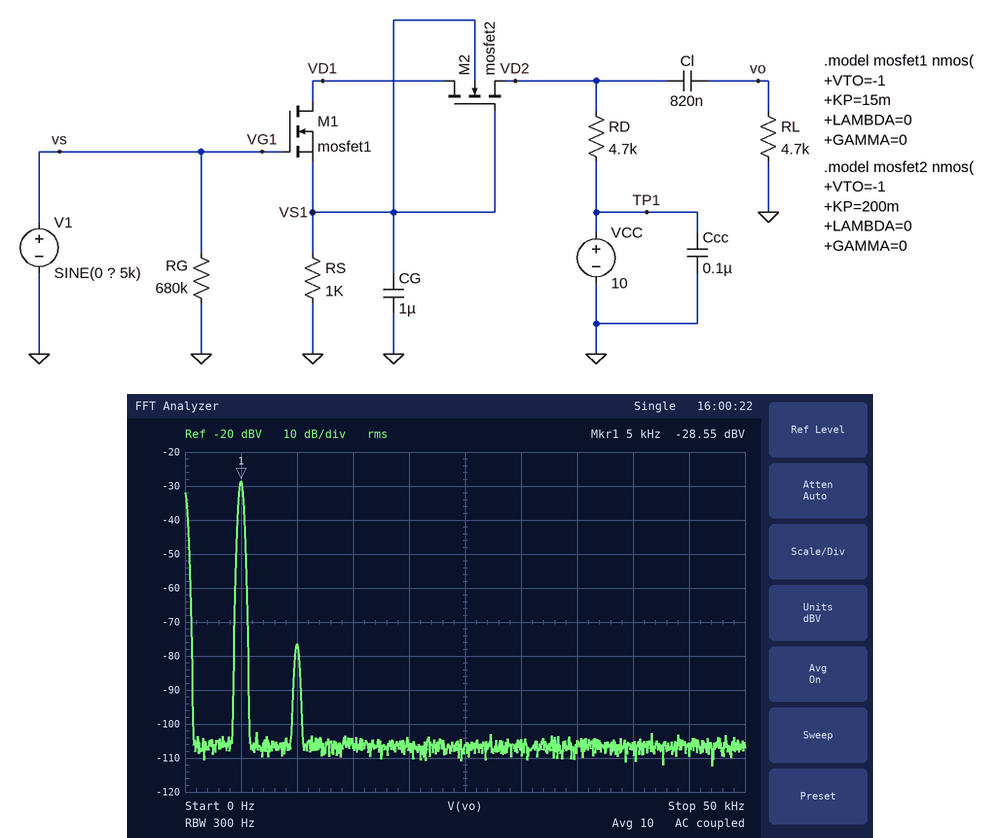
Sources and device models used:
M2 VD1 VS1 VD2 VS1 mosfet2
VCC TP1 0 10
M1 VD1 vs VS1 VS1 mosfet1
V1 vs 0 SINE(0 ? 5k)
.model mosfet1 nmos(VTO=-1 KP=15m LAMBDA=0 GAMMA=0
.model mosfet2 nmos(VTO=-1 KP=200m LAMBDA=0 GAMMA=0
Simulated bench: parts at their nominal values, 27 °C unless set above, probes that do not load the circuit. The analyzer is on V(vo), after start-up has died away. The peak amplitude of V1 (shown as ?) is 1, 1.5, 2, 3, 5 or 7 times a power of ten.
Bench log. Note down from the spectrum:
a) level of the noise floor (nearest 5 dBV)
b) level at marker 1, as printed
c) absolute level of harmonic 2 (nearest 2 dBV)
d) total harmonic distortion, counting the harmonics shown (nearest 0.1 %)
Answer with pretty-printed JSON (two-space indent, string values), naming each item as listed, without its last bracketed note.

{
  "level of the noise floor": "-105 dBV",
  "level at marker 1, as printed": "-28.55 dBV",
  "absolute level of harmonic 2": "-76 dBV",
  "total harmonic distortion, counting the harmonics shown": "0.4 %"
}
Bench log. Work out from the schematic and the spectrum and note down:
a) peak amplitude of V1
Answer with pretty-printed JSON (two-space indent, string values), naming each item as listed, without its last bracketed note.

{
  "peak amplitude of V1": "5 mV"
}
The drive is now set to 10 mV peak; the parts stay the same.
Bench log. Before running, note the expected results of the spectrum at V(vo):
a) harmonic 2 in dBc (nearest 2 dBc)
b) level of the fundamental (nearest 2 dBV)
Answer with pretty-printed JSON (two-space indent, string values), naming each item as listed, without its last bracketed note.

{
  "harmonic 2 in dBc": "-42 dBc",
  "level of the fundamental": "-22 dBV"
}
